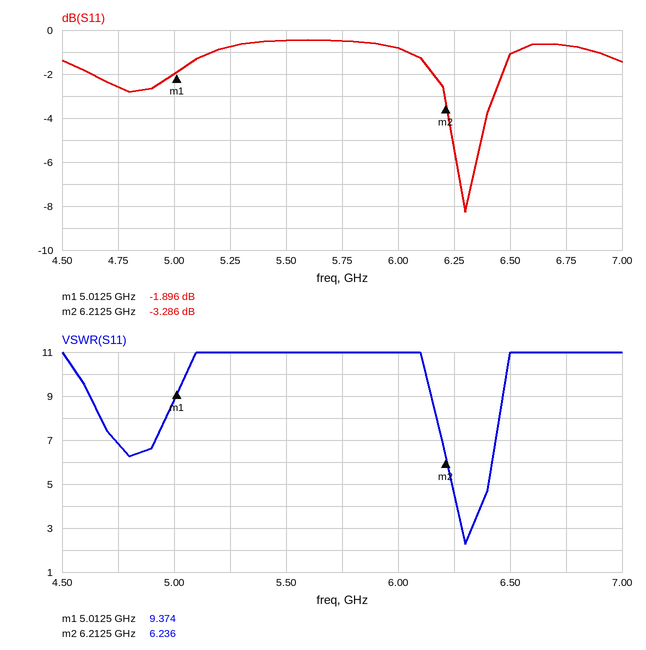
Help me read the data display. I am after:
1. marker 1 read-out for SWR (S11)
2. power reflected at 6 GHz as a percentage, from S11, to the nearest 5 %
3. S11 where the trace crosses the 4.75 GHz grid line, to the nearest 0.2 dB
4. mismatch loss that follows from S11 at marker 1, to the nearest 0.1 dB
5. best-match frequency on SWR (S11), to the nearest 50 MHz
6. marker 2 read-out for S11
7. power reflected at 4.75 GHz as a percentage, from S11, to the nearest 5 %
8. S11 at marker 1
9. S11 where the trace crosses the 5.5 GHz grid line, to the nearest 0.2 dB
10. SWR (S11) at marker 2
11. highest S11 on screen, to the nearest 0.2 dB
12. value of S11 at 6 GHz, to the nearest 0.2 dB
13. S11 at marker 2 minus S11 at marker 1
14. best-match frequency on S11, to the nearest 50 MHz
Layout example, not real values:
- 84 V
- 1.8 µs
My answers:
- 9.374
- 85 %
- -2.6 dB
- 4.5 dB
- 6.30 GHz
- -3.286 dB
- 55 %
- -1.896 dB
- -0.4 dB
- 6.236
- -0.4 dB
- -0.8 dB
- -1.390 dB
- 6.30 GHz
